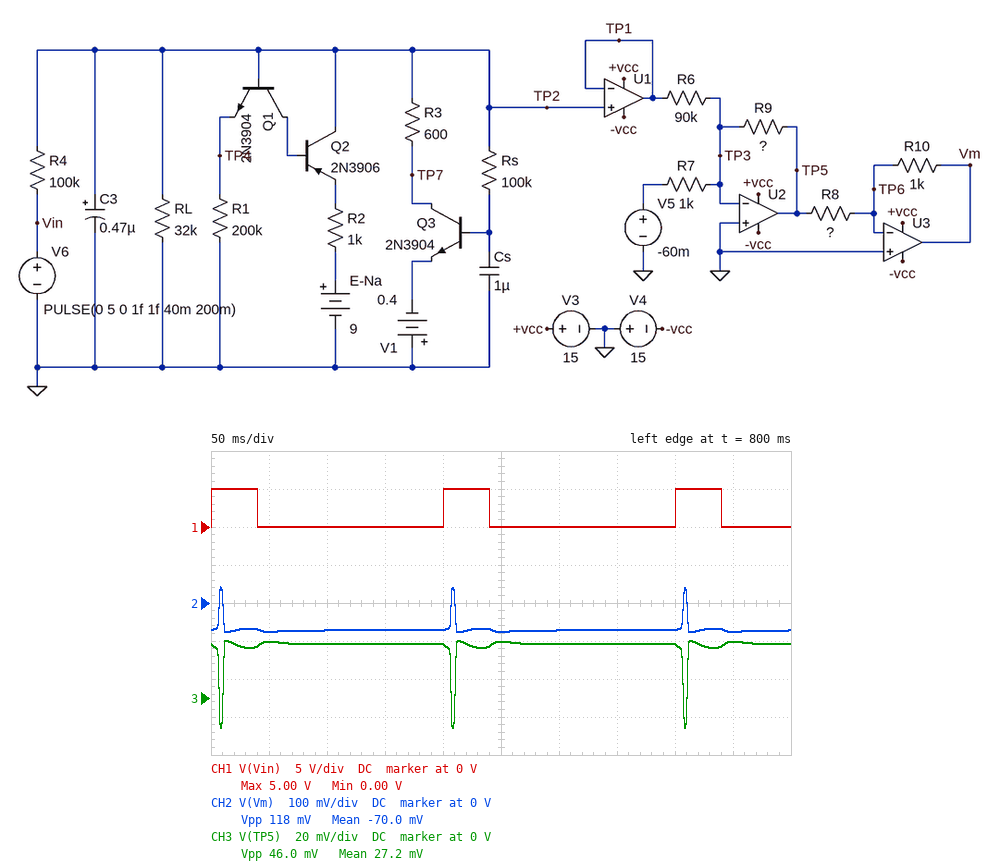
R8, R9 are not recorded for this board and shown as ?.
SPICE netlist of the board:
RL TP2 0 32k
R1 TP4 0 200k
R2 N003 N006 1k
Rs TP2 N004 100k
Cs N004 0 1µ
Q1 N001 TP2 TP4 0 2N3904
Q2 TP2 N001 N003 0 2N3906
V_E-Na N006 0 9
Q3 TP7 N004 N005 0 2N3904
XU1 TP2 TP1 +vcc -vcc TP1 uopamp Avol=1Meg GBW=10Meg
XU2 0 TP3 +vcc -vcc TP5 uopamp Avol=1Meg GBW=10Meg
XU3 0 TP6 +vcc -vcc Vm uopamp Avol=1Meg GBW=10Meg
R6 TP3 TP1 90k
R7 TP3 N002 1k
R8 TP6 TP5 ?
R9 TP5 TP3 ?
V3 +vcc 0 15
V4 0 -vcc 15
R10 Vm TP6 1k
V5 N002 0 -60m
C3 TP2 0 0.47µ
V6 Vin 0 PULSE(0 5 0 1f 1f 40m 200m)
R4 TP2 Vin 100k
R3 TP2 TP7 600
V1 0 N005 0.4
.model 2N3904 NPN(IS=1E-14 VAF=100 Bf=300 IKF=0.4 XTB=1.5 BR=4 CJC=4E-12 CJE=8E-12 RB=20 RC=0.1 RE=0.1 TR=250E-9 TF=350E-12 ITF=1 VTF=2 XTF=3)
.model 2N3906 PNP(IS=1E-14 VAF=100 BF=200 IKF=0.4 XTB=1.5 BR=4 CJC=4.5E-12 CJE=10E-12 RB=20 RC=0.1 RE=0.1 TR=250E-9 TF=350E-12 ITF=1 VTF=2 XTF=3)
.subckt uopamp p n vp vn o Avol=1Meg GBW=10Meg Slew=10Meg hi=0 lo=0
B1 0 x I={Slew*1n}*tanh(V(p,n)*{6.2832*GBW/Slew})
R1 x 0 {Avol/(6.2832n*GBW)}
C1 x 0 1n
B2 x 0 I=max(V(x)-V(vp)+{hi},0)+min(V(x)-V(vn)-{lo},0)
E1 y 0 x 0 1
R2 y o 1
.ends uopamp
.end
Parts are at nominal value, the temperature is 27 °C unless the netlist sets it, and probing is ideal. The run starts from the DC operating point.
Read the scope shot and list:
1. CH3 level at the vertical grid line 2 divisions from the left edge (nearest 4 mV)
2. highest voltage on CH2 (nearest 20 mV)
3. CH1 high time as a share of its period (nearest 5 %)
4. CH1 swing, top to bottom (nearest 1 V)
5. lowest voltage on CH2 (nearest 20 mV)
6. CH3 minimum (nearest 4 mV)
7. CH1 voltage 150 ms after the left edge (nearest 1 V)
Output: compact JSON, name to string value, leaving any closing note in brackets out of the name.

{"CH3 level at the vertical grid line 2 divisions from the left edge": "28 mV", "highest voltage on CH2": "40 mV", "CH1 high time as a share of its period": "20 %", "CH1 swing, top to bottom": "5 V", "lowest voltage on CH2": "-80 mV", "CH3 minimum": "-16 mV", "CH1 voltage 150 ms after the left edge": "0 V"}
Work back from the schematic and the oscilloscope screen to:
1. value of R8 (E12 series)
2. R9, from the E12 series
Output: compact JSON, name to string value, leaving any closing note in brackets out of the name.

{"value of R8": "390 Ω", "R9, from the E12 series": "470 Ω"}
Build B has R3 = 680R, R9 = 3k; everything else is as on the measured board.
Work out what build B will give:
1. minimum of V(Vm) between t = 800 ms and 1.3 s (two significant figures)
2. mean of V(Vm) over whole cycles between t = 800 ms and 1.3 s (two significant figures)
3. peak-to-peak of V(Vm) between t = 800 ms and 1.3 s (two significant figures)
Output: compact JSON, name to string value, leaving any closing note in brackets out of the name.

{"minimum of V(Vm) between t = 800 ms and 1.3 s": "-490 mV", "mean of V(Vm) over whole cycles between t = 800 ms and 1.3 s": "-450 mV", "peak-to-peak of V(Vm) between t = 800 ms and 1.3 s": "750 mV"}
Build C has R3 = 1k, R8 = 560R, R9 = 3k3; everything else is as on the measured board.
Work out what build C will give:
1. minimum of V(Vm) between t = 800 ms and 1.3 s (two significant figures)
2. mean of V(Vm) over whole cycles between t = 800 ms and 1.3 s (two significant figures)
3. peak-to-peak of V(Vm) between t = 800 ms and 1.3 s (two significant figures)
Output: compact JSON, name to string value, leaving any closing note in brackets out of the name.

{"minimum of V(Vm) between t = 800 ms and 1.3 s": "-370 mV", "mean of V(Vm) over whole cycles between t = 800 ms and 1.3 s": "-340 mV", "peak-to-peak of V(Vm) between t = 800 ms and 1.3 s": "570 mV"}
